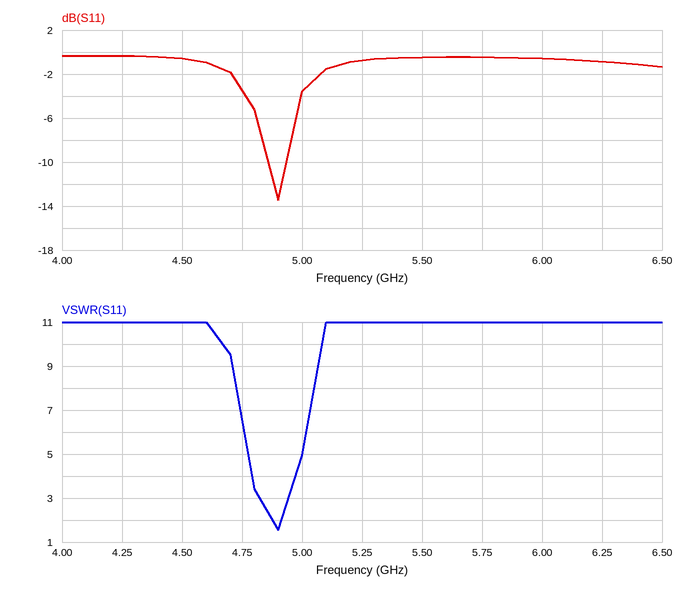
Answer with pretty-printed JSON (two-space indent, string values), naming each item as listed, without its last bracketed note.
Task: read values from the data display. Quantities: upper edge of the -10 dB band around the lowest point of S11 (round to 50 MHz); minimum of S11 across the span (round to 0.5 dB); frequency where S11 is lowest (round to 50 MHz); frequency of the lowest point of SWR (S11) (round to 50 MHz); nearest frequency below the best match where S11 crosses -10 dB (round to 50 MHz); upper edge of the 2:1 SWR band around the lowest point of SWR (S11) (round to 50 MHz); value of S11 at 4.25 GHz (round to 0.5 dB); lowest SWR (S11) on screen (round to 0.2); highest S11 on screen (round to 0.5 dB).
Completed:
{
  "upper edge of the -10 dB band around the lowest point of S11": "4.95 GHz",
  "minimum of S11 across the span": "-13.5 dB",
  "frequency where S11 is lowest": "4.90 GHz",
  "frequency of the lowest point of SWR (S11)": "4.90 GHz",
  "nearest frequency below the best match where S11 crosses -10 dB": "4.85 GHz",
  "upper edge of the 2:1 SWR band around the lowest point of SWR (S11)": "4.90 GHz",
  "value of S11 at 4.25 GHz": "-0.5 dB",
  "lowest SWR (S11) on screen": "1.6",
  "highest S11 on screen": "-0.5 dB"
}
